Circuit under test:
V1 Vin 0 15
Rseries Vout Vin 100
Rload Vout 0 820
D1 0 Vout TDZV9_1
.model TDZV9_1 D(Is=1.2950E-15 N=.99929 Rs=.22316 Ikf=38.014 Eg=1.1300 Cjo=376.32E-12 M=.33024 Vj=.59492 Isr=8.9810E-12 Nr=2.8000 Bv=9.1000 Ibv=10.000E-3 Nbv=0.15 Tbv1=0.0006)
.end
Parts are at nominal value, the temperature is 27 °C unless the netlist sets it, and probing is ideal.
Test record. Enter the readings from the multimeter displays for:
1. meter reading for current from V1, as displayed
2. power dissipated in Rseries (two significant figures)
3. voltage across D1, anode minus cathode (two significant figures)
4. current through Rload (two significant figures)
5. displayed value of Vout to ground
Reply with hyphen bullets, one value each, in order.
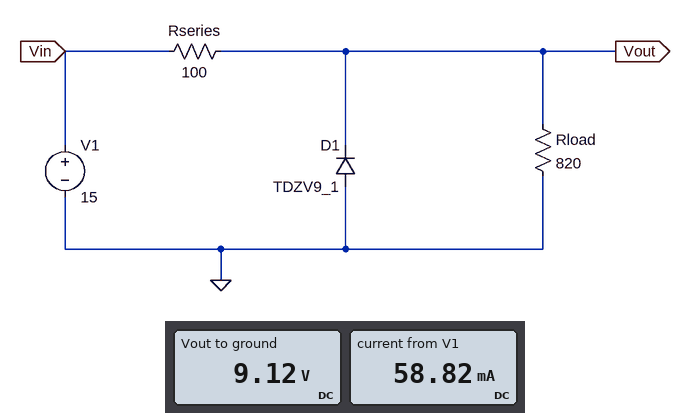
- 58.82 mA
- 350 mW
- -9.1 V
- 11 mA
- 9.12 V
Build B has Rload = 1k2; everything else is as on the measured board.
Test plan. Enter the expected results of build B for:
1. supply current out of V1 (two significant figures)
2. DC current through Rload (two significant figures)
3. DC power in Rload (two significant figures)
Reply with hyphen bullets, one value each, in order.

- 59 mA
- 7.6 mA
- 69 mW
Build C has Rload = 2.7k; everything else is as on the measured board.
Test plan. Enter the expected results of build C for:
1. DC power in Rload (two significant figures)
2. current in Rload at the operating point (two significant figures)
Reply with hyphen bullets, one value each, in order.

- 31 mW
- 3.4 mA
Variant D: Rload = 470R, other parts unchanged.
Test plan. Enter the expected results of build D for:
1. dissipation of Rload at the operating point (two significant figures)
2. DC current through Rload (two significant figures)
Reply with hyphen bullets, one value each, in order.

- 180 mW
- 19 mA
